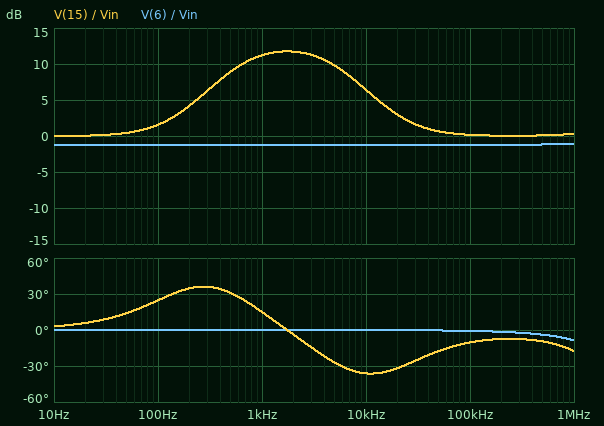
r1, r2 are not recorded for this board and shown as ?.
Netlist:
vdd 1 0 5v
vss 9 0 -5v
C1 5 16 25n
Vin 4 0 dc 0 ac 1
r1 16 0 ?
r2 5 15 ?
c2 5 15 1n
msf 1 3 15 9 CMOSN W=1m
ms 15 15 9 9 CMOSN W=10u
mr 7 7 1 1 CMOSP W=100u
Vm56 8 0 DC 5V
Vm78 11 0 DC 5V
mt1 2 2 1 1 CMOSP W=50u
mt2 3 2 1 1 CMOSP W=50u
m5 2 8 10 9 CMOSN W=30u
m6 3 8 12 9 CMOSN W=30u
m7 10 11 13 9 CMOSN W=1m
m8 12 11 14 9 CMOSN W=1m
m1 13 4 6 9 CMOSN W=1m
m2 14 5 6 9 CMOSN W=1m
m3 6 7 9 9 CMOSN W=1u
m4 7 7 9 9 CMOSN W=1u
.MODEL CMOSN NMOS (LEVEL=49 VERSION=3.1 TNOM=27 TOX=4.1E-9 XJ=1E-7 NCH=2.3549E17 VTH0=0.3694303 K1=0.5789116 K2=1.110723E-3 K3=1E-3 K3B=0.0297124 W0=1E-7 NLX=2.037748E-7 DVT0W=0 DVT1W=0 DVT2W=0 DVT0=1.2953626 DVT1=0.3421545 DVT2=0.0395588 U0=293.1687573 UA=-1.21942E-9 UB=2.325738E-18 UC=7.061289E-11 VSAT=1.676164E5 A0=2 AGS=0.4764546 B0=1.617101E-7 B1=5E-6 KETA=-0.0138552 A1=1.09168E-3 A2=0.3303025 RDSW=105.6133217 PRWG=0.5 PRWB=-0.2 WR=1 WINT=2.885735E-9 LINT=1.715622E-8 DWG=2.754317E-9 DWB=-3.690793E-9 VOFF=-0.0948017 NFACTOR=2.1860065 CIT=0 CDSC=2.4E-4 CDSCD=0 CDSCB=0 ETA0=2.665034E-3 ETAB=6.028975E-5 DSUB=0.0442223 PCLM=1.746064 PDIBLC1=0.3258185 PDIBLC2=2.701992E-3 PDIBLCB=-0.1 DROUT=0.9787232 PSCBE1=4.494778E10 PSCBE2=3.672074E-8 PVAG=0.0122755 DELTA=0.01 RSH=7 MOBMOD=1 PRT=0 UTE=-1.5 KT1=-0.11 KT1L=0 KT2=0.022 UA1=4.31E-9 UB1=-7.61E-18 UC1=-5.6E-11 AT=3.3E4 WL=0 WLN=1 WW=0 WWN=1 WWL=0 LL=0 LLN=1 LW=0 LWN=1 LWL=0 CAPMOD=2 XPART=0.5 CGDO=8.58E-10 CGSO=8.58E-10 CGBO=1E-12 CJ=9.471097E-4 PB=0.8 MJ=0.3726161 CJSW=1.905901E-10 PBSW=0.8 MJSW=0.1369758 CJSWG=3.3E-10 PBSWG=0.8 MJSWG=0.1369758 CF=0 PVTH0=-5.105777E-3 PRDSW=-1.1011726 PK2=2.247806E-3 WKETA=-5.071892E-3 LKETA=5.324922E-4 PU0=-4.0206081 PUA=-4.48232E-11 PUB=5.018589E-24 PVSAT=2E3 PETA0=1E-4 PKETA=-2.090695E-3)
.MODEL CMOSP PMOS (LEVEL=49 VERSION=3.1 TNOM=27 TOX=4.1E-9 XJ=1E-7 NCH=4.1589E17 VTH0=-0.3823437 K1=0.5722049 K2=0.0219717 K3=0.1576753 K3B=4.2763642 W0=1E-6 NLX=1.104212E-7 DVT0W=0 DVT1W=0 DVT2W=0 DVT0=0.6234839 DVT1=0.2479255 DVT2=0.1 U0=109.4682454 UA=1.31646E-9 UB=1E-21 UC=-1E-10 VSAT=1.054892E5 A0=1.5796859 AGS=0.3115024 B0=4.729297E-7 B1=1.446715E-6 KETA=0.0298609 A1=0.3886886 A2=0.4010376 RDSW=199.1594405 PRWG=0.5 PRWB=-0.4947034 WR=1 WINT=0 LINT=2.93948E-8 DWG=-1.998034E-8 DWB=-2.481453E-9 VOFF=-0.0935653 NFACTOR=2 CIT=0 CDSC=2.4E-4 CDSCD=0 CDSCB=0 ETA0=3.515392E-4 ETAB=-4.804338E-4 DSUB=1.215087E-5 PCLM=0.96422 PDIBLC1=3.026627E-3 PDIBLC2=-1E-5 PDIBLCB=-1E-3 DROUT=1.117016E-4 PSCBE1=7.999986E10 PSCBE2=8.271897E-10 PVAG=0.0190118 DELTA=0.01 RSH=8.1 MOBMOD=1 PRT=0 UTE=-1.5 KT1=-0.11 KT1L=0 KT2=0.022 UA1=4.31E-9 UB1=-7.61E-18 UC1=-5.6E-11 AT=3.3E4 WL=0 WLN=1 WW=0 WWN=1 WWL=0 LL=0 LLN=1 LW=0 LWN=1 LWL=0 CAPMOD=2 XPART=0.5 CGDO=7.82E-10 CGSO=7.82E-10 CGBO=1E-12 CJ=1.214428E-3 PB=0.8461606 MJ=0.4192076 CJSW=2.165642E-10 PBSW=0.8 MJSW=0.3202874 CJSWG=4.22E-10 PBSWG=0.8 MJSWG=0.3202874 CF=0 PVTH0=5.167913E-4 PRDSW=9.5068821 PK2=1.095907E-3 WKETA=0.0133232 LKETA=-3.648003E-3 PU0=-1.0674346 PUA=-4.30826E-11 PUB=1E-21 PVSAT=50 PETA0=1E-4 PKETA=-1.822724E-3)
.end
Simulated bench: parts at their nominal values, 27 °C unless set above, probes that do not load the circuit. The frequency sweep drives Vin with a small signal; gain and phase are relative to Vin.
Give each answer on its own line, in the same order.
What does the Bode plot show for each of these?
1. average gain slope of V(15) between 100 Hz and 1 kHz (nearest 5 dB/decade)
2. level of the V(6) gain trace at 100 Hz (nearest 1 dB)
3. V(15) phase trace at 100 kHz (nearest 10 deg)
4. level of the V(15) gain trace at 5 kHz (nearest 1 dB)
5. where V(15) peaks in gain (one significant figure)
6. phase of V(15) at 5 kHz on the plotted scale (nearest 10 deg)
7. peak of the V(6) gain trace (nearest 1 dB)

10 dB/decade
-1 dB
-10 deg
10 dB
2 kHz
-30 deg
-1 dB
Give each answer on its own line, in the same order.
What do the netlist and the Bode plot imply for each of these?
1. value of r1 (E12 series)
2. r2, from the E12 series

10 kΩ
33 kΩ
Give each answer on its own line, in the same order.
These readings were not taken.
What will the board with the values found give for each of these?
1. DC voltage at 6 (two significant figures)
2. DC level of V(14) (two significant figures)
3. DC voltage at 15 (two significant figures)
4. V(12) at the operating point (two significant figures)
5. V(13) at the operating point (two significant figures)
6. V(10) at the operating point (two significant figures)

-1.1 V
1.5 V
4.7 mV
1.5 V
3.1 V
3.1 V
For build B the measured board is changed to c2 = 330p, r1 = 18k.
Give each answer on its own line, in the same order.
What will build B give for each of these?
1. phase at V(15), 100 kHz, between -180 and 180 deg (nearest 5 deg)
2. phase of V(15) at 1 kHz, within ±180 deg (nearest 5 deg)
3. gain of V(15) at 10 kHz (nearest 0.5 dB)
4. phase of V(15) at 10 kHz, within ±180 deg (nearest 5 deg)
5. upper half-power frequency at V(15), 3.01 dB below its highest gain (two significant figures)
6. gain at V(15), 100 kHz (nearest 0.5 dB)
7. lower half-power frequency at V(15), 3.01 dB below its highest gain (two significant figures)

-15 deg
10 deg
7.5 dB
-20 deg
18 kHz
0.5 dB
290 Hz
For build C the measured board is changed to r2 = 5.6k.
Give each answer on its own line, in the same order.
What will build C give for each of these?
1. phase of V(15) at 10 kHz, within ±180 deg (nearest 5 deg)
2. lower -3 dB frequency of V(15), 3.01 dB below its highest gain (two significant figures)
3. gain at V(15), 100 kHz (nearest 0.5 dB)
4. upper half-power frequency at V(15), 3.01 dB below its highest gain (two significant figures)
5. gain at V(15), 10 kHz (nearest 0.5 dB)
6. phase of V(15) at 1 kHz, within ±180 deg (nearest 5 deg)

-5 deg
250 Hz
0.5 dB
73 kHz
3.5 dB
10 deg
